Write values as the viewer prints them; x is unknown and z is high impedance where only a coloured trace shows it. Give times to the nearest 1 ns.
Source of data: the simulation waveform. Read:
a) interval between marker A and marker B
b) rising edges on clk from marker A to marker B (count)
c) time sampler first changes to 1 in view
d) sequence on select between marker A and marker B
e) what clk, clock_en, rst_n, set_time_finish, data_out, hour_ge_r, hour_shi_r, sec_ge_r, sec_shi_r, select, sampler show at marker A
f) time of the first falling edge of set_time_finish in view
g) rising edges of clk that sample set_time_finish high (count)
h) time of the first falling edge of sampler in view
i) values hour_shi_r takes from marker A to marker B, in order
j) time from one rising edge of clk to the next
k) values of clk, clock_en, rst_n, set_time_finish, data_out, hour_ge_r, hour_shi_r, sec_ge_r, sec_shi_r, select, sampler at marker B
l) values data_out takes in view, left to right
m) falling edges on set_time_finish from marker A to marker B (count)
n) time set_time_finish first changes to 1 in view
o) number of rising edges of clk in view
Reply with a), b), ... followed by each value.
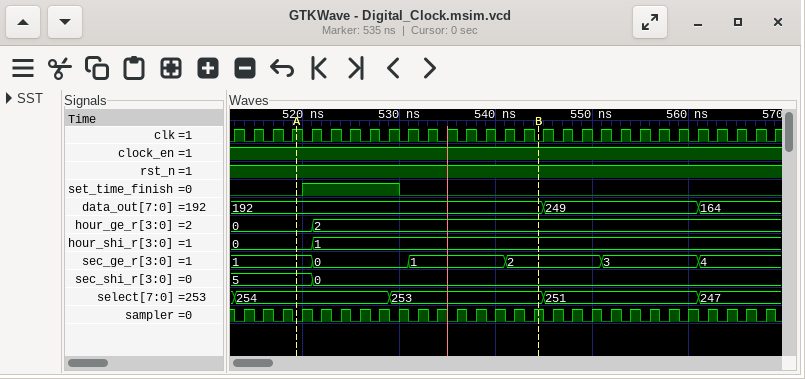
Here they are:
a) 25 ns
b) 12
c) 514 ns
d) 254, 253
e) clk=1, clock_en=1, rst_n=1, set_time_finish=0, data_out=192, hour_ge_r=0, hour_shi_r=0, sec_ge_r=1, sec_shi_r=5, select=254, sampler=0
f) 530 ns
g) 5
h) 513 ns
i) 0, 1
j) 2 ns
k) clk=0, clock_en=1, rst_n=1, set_time_finish=0, data_out=192, hour_ge_r=2, hour_shi_r=1, sec_ge_r=2, sec_shi_r=0, select=253, sampler=1
l) 192, 249, 164
m) 1
n) 520 ns
o) 29
